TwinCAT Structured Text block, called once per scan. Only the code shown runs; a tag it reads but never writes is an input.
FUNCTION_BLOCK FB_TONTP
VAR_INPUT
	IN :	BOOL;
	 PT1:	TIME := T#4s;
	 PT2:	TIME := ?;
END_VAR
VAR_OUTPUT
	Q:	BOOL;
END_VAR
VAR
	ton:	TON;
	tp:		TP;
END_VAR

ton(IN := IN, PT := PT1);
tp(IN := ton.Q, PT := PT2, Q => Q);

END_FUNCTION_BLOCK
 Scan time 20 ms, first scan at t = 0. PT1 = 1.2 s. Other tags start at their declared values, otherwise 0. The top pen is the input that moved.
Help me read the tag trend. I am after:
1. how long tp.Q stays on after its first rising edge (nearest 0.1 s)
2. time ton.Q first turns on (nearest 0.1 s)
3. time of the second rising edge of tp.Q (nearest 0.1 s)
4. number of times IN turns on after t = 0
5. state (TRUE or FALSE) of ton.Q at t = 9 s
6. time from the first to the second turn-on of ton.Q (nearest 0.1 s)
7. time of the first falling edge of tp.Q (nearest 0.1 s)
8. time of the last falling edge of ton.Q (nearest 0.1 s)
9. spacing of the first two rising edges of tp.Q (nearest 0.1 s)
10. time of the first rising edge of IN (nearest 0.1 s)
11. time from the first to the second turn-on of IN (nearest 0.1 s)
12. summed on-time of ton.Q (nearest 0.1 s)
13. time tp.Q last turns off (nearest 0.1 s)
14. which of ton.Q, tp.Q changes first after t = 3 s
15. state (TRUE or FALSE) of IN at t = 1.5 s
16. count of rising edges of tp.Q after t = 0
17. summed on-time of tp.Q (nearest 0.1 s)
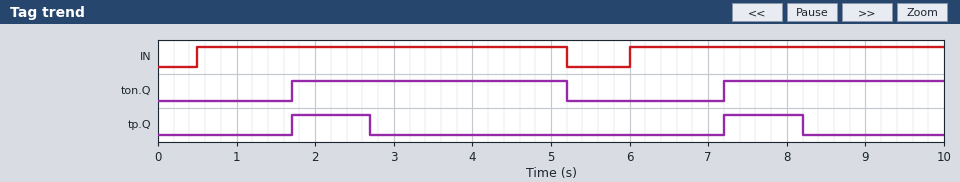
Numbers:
1.0 s
1.7 s
7.2 s
2
TRUE
5.5 s
2.7 s
5.2 s
5.5 s
0.5 s
5.5 s
6.3 s
8.2 s
ton.Q
TRUE
2
2.0 s
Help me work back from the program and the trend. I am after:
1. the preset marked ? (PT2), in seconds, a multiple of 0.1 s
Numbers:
1.0 s
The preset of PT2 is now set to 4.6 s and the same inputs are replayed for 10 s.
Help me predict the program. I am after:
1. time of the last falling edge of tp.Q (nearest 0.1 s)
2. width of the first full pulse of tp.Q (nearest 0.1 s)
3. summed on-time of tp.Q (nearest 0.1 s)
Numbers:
6.3 s
4.6 s
7.4 s
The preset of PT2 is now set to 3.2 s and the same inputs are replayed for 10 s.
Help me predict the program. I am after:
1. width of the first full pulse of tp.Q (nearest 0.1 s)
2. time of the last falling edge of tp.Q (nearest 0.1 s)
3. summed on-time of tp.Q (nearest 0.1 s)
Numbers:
3.2 s
4.9 s
6.0 s
